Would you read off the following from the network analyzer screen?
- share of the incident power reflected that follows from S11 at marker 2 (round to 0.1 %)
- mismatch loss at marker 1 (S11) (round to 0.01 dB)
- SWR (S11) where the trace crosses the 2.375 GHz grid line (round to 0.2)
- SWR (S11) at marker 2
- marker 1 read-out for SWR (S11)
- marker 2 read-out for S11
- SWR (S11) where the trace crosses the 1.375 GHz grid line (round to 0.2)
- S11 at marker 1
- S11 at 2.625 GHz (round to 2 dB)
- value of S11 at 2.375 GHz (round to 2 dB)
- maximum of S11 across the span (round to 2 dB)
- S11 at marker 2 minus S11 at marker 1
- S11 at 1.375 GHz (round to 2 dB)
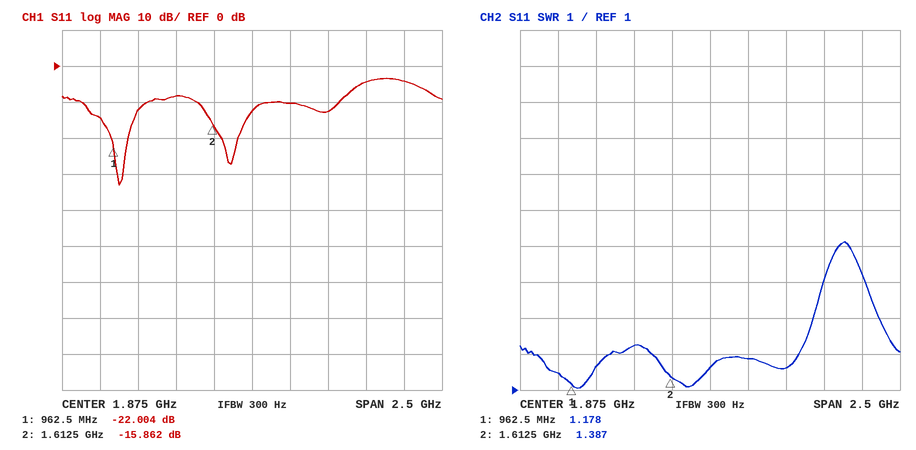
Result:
2.6 %
0.03 dB
1.6
1.387
1.178
-15.862 dB
2.2
-22.004 dB
-4 dB
-12 dB
-4 dB
6.142 dB
-8 dB
